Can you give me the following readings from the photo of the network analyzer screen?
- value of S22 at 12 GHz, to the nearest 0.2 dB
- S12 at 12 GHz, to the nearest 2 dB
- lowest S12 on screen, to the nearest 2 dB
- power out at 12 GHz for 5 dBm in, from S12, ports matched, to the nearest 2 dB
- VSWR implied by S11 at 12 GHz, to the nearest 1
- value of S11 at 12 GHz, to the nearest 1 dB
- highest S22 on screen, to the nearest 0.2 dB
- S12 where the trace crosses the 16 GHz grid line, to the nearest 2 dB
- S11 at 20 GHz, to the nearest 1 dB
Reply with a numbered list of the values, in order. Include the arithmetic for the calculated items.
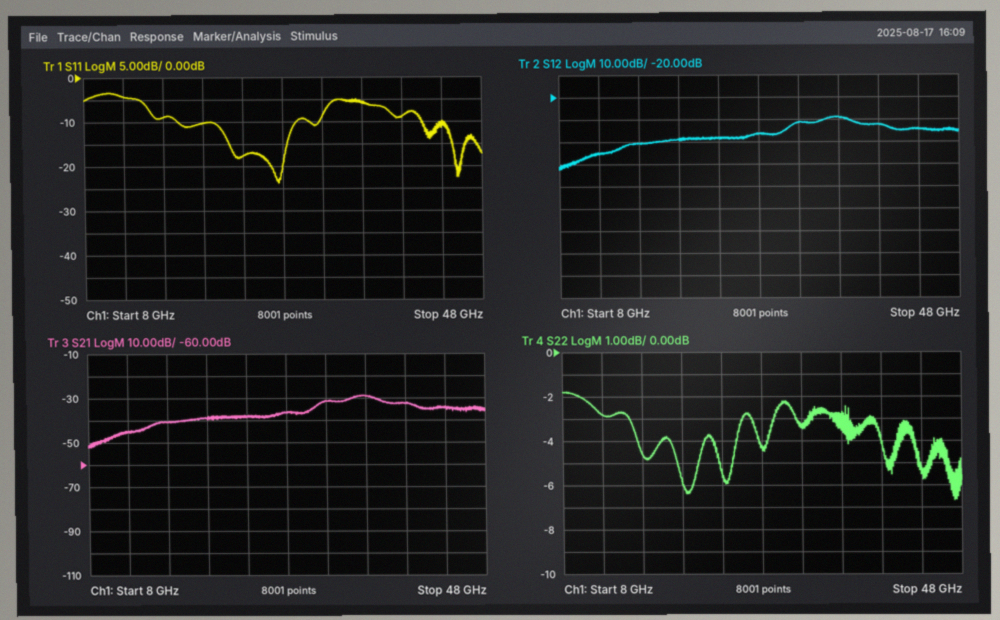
1. -2.8 dB
2. -46 dB
3. -52 dB
4. 5 dBm + (-46 dB) = -40 dBm
5. |Γ| = 10^(-4/20) = 0.6310; VSWR = (1 + 0.6310)/(1 − 0.6310) ≈ 4
6. -4 dB
7. -1.8 dB
8. -40 dB
9. -10 dB
